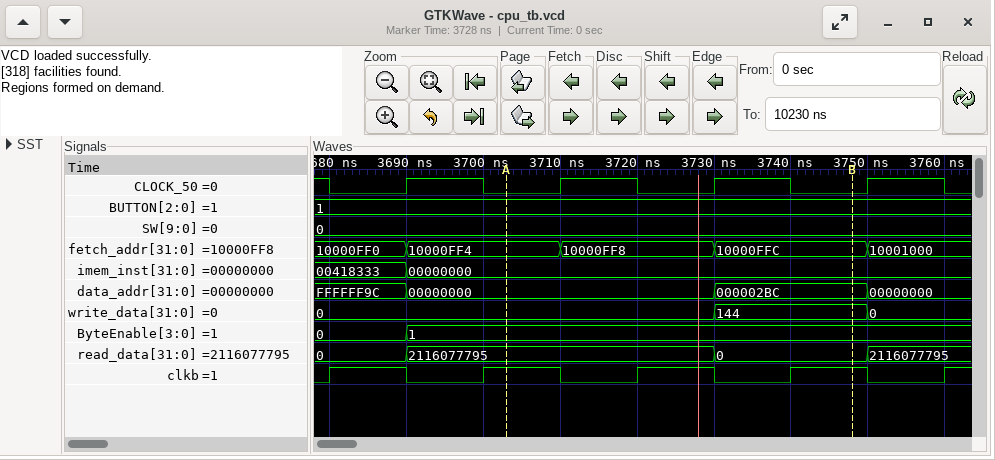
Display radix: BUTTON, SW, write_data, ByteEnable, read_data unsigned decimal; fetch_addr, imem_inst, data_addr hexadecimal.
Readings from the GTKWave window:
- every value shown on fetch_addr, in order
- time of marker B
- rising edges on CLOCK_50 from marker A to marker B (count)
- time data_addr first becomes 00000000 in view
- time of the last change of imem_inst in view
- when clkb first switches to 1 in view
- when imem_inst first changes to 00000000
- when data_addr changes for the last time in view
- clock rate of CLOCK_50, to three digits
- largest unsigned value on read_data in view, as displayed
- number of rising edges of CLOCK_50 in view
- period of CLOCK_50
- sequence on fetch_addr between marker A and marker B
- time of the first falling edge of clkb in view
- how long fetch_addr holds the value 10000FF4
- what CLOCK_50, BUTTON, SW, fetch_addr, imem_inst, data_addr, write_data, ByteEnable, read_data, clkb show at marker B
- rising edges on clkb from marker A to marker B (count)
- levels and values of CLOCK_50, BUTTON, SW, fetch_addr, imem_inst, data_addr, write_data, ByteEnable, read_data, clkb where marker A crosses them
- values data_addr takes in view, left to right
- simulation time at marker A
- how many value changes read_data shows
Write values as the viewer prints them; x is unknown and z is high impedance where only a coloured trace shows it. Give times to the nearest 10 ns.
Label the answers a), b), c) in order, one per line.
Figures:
a) 10000FF0, 10000FF4, 10000FF8, 10000FFC, 10001000
b) 3750 ns
c) 2
d) 3690 ns
e) 3690 ns
f) 3680 ns
g) 3690 ns
h) 3750 ns
i) 50.0 MHz
j) 2116077795
k) 4
l) 20 ns
m) 10000FF4, 10000FF8, 10000FFC
n) 3690 ns
o) 20 ns
p) CLOCK_50=0, BUTTON=1, SW=0, fetch_addr=10000FFC, imem_inst=00000000, data_addr=000002BC, write_data=144, ByteEnable=1, read_data=0, clkb=1
q) 2
r) CLOCK_50=0, BUTTON=1, SW=0, fetch_addr=10000FF4, imem_inst=00000000, data_addr=00000000, write_data=0, ByteEnable=1, read_data=2116077795, clkb=1
s) FFFFFF9C, 00000000, 000002BC, 00000000
t) 3700 ns
u) 3
